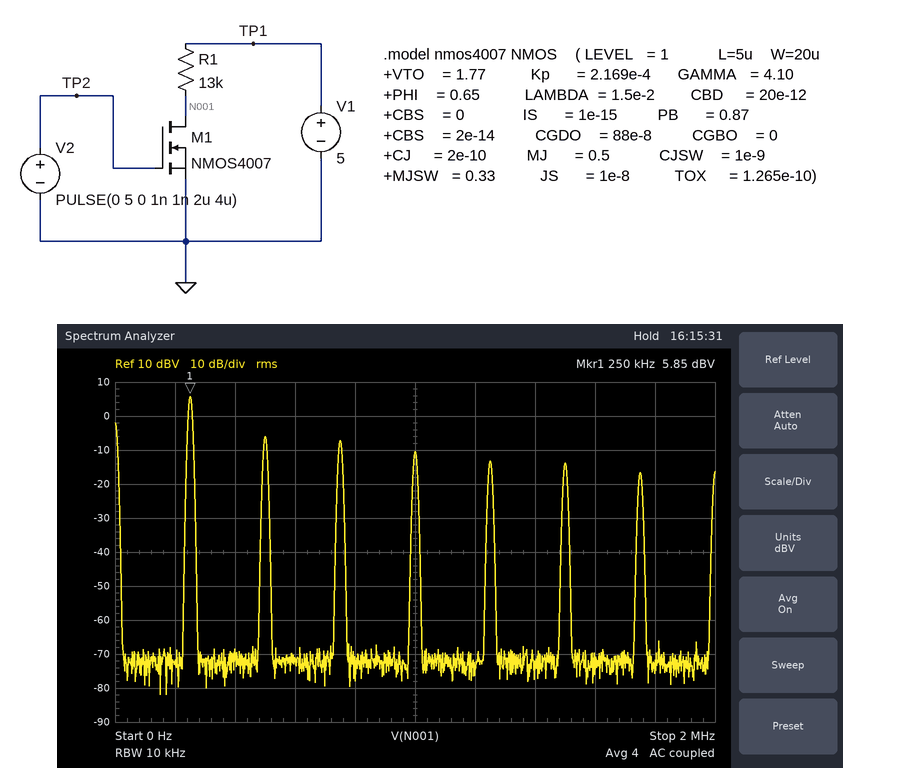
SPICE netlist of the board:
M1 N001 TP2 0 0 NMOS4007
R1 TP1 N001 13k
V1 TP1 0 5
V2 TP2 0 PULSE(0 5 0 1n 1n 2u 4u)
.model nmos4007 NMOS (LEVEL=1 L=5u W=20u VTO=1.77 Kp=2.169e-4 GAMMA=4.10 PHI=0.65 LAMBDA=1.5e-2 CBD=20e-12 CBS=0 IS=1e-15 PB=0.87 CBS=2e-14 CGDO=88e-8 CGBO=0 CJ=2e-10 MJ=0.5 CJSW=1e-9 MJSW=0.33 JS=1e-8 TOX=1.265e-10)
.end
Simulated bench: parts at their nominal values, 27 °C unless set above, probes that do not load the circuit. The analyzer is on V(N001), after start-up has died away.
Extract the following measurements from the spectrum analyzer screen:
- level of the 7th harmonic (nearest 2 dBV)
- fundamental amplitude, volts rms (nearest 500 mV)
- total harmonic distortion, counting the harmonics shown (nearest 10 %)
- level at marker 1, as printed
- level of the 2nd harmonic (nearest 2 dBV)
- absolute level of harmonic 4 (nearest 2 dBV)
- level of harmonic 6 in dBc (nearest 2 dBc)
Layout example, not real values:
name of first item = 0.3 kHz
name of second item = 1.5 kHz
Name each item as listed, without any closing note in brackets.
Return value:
level of the 7th harmonic = -16 dBV
fundamental amplitude, volts rms = 2.0 V
total harmonic distortion, counting the harmonics shown = 40 %
level at marker 1, as printed = 5.85 dBV
level of the 2nd harmonic = -6 dBV
absolute level of harmonic 4 = -10 dBV
level of harmonic 6 in dBc = -20 dBc
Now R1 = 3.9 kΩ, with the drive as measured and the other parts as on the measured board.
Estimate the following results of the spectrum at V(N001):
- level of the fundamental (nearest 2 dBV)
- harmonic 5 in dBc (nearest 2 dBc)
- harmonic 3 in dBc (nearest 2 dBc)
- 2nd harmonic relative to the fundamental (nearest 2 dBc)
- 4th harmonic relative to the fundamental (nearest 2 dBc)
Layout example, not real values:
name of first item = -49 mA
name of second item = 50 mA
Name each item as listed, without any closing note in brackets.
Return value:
level of the fundamental = 6 dBV
harmonic 5 in dBc = -16 dBc
harmonic 3 in dBc = -10 dBc
2nd harmonic relative to the fundamental = -22 dBc
4th harmonic relative to the fundamental = -22 dBc
